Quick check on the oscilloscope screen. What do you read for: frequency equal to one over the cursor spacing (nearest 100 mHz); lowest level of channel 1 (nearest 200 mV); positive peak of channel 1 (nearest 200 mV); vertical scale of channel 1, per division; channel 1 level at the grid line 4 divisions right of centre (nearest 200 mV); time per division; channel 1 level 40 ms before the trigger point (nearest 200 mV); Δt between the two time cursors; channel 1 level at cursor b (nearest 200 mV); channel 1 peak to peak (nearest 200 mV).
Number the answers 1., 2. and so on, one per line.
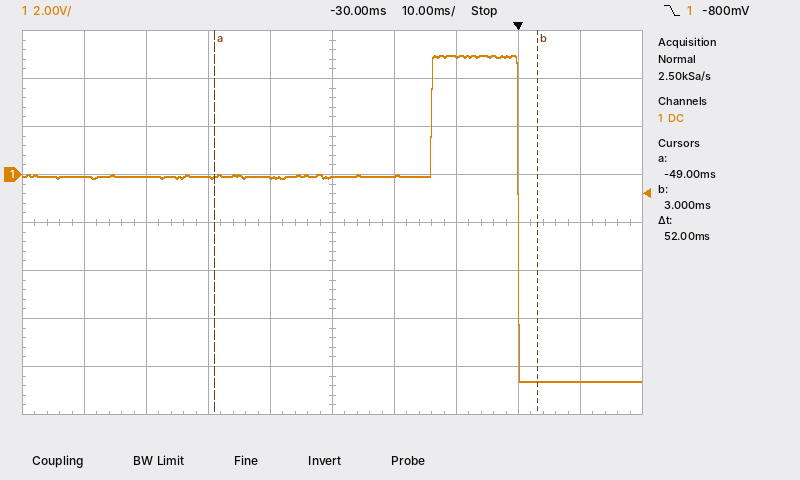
1. 19.2 Hz
2. -8.6 V
3. 5.0 V
4. 2 V
5. -8.6 V
6. 10 ms
7. -200 mV
8. 52 ms
9. -8.6 V
10. 13.6 V
